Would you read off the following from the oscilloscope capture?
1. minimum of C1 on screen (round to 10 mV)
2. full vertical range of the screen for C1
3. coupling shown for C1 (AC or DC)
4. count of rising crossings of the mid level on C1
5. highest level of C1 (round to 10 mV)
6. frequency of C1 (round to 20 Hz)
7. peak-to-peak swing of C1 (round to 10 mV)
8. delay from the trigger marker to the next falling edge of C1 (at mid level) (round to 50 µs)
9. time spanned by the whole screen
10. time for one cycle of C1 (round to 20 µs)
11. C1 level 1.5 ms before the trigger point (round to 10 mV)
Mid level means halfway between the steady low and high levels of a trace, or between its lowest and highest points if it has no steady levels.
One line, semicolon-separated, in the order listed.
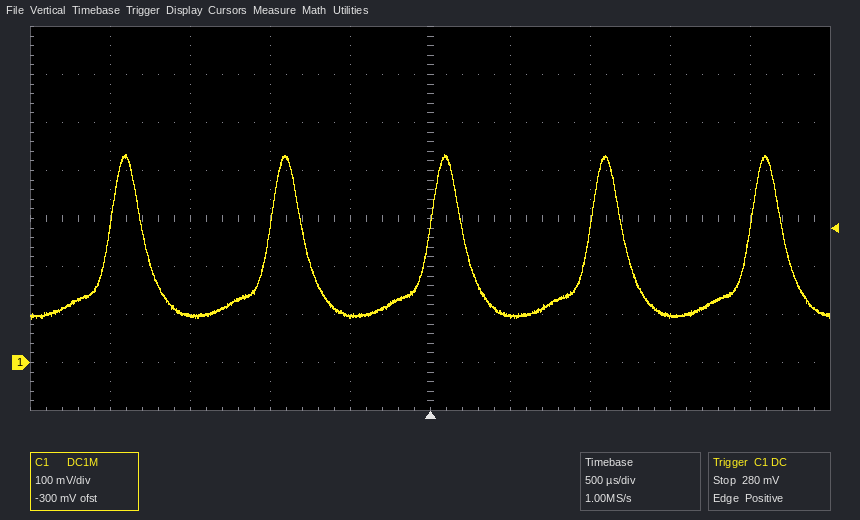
90 mV; 800 mV; DC; 5; 430 mV; 1.00 kHz; 340 mV; 200 µs; 5 ms; 1.00 ms; 100 mV
